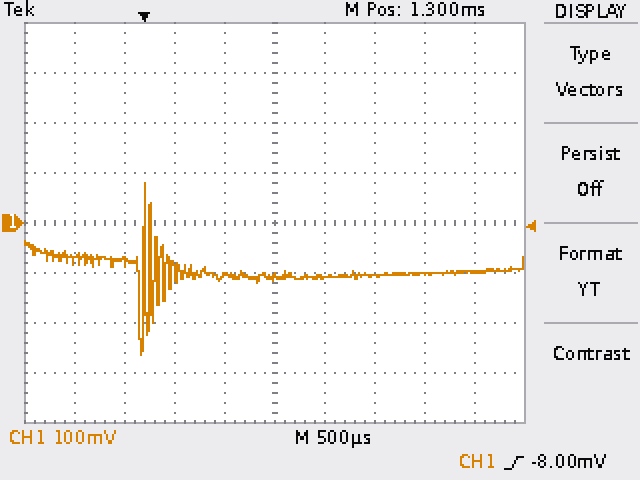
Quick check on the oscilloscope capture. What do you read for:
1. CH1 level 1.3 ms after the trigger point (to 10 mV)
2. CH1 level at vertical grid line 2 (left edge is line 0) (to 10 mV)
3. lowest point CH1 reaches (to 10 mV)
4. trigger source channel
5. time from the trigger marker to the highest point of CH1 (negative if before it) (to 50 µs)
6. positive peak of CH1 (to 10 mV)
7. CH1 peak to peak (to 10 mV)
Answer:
-110 mV
-80 mV
-260 mV
CH1
0 µs
80 mV
340 mV
